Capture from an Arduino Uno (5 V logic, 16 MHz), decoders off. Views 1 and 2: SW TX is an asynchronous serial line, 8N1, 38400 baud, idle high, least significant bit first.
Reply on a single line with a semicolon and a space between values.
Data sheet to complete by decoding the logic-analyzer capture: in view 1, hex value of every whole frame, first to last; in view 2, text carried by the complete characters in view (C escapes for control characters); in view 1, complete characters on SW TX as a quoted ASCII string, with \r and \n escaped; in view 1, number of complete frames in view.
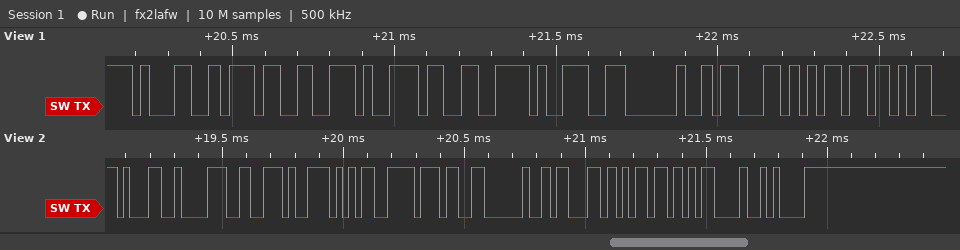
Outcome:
0x31 0x37 0x2E 0x33 0x39 0x20 0x63 0x6D; "18.57 cm\r\n"; "17.39 cm"; 8
